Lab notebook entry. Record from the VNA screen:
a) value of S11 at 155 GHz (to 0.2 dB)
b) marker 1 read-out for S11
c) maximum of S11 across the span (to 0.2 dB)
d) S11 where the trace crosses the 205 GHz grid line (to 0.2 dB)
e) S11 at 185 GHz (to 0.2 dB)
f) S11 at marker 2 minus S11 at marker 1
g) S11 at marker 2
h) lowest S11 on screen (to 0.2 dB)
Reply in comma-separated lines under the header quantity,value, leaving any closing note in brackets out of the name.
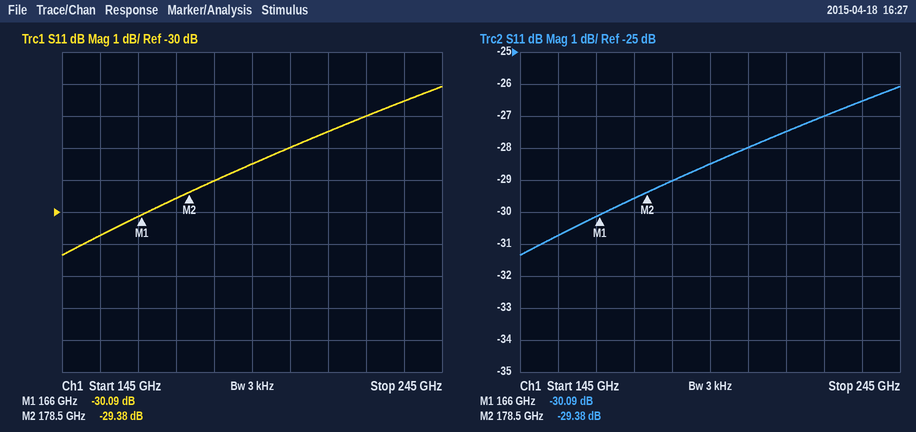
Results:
quantity,value
value of S11 at 155 GHz,-30.8 dB
marker 1 read-out for S11,-30.09 dB
maximum of S11 across the span,-26.0 dB
S11 where the trace crosses the 205 GHz grid line,-28.0 dB
S11 at 185 GHz,-29.0 dB
S11 at marker 2 minus S11 at marker 1,0.71 dB
S11 at marker 2,-29.38 dB
lowest S11 on screen,-31.4 dB
